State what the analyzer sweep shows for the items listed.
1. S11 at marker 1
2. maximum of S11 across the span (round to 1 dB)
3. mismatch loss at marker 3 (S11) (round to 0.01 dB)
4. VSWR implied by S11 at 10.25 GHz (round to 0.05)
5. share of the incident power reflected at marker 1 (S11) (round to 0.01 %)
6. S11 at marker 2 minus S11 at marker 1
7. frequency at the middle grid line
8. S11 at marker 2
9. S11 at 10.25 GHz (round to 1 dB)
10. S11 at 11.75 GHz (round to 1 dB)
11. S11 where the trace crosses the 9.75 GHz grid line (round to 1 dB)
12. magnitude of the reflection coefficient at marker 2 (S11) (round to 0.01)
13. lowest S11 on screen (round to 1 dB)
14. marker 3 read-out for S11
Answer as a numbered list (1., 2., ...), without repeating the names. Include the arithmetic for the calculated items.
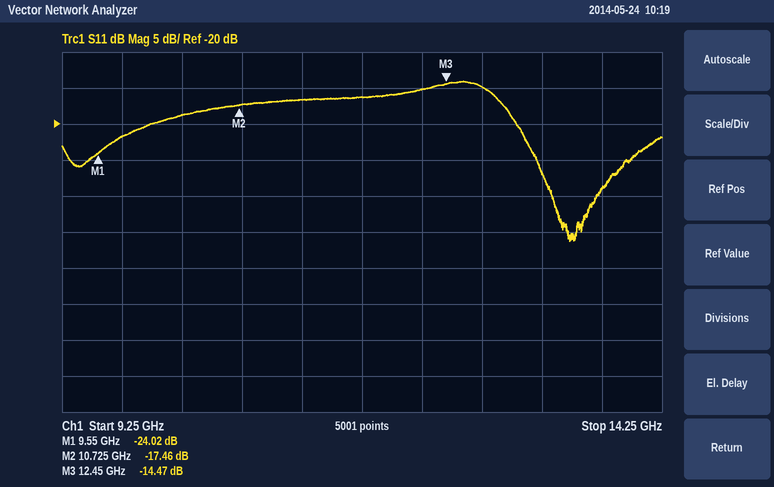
1. -24.02 dB
2. -14 dB
3. −10 log10(1 − 10^(-14.47/10)) ≈ 0.16 dB
4. |Γ| = 10^(-19/20) = 0.1122; VSWR = (1 + 0.1122)/(1 − 0.1122) ≈ 1.25
5. 10^(-24.02/10) ≈ 0.40 %
6. -17.46 − (-24.02) = 6.56 dB
7. 11.75 GHz
8. -17.46 dB
9. -19 dB
10. -16 dB
11. -22 dB
12. 10^(-17.46/20) ≈ 0.13
13. -36 dB
14. -14.47 dB
